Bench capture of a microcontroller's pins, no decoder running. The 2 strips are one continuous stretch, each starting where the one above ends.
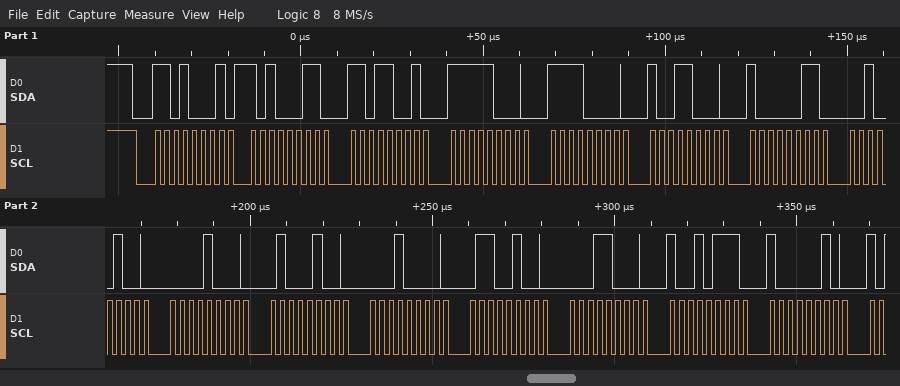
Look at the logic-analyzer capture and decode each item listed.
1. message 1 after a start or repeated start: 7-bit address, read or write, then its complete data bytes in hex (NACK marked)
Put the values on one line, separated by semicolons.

0x68 read: A3 D9 F8 F0 98 83 24 08 44 10 64 18 97 82
